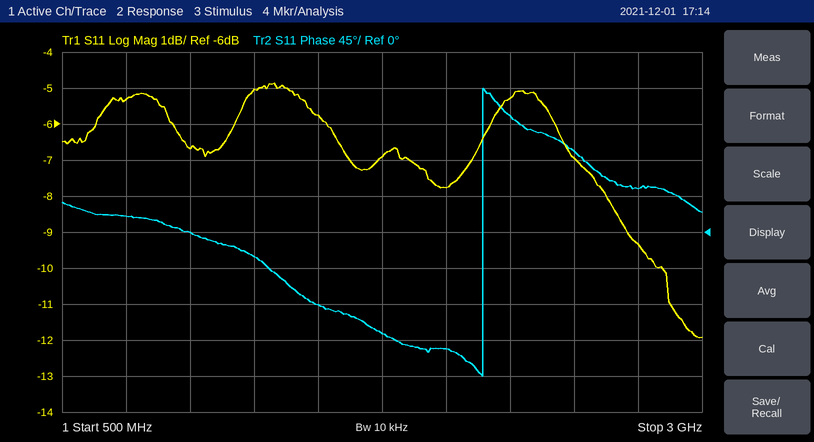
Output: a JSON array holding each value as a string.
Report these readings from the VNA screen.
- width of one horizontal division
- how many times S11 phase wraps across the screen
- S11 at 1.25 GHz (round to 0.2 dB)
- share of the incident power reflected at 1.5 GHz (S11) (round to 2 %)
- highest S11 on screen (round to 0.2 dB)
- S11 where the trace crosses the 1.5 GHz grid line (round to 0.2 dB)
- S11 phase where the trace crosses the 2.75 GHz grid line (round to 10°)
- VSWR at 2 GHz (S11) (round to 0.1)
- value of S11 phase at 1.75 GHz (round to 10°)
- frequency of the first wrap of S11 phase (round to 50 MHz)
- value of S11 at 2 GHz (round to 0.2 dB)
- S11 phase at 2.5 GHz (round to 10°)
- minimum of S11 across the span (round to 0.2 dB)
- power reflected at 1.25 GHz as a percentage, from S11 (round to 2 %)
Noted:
["250 MHz", "1", "-5.0 dB", "26 %", "-4.8 dB", "-5.8 dB", "50°", "2.4", "-130°", "2.15 GHz", "-7.8 dB", "100°", "-12.0 dB", "32 %"]
